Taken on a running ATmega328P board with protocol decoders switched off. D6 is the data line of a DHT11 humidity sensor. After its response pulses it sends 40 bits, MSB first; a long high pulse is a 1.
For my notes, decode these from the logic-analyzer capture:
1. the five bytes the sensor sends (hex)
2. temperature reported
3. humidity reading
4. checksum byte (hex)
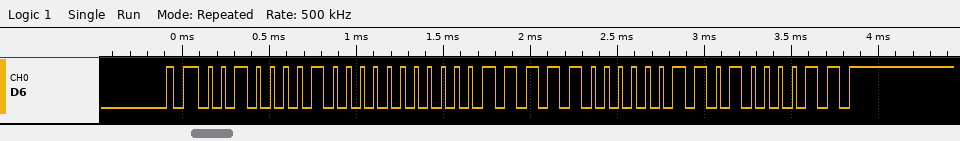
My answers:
21 00 1F 03 43
31.3 °C
33 %
0x43
